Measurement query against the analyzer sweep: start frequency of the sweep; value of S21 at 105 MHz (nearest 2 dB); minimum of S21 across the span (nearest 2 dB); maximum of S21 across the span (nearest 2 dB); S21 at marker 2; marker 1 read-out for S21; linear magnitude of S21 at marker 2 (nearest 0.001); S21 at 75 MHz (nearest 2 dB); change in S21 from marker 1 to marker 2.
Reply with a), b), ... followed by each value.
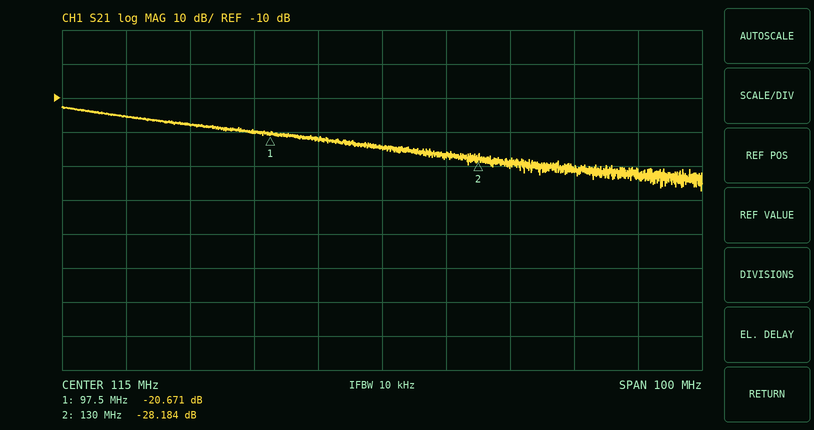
a) 65 MHz
b) -22 dB
c) -38 dB
d) -12 dB
e) -28.184 dB
f) -20.671 dB
g) 0.039
h) -16 dB
i) -7.513 dB
